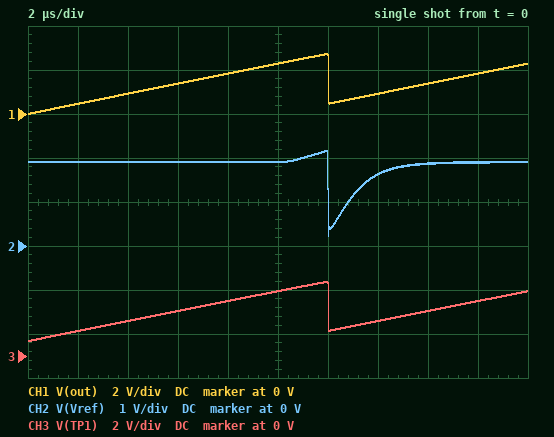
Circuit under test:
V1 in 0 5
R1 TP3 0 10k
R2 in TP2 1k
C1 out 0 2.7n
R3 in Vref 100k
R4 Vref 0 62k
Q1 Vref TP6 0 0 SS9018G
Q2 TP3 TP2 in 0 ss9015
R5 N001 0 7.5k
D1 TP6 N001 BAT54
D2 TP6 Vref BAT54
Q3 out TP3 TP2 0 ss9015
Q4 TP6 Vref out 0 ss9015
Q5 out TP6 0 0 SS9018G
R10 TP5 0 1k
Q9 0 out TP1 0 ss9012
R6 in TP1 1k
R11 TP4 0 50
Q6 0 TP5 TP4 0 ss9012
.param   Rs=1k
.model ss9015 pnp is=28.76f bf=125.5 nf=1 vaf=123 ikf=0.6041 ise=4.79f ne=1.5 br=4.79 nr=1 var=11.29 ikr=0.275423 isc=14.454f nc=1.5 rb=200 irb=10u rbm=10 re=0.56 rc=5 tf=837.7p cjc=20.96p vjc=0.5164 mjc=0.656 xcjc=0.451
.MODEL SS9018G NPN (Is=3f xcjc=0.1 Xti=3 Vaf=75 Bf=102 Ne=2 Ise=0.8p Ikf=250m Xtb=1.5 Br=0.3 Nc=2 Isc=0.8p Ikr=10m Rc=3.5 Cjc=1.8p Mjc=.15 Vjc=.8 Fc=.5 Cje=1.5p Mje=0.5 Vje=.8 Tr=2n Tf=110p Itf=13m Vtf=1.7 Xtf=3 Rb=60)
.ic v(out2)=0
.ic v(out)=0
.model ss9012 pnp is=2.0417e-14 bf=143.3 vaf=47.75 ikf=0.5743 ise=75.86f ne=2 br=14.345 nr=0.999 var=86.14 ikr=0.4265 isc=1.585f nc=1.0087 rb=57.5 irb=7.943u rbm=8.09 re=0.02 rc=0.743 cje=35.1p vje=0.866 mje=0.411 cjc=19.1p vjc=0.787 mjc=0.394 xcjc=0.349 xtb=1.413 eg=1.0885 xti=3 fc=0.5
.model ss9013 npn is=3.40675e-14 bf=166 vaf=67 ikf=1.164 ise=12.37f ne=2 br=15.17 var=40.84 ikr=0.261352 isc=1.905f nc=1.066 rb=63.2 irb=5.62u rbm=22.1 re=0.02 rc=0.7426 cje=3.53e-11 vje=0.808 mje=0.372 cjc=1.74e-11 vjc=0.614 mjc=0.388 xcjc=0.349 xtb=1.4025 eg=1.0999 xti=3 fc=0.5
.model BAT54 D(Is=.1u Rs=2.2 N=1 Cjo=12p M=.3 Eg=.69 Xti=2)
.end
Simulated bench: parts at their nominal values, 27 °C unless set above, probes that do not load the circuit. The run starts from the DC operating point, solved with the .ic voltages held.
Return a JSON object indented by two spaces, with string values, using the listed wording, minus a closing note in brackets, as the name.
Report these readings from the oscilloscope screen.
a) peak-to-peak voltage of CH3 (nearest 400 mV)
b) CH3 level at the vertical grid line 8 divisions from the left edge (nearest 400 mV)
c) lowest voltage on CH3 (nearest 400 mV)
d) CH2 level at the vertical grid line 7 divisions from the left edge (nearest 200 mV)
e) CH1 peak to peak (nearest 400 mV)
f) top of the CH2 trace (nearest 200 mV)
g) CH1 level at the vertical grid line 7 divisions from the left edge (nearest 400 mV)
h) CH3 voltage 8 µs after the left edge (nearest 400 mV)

{
  "peak-to-peak voltage of CH3": "2.8 V",
  "CH3 level at the vertical grid line 8 divisions from the left edge": "2.0 V",
  "lowest voltage on CH3": "800 mV",
  "CH2 level at the vertical grid line 7 divisions from the left edge": "1.6 V",
  "CH1 peak to peak": "2.8 V",
  "top of the CH2 trace": "2.2 V",
  "CH1 level at the vertical grid line 7 divisions from the left edge": "800 mV",
  "CH3 voltage 8 µs after the left edge": "2.4 V"
}
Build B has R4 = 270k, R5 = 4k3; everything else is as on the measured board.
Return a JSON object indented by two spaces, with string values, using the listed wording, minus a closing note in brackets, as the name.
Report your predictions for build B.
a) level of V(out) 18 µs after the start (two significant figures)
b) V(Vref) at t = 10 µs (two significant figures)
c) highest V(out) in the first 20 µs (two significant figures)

{
  "level of V(out) 18 µs after the start": "4.1 V",
  "V(Vref) at t = 10 µs": "3.6 V",
  "highest V(out) in the first 20 µs": "4.4 V"
}
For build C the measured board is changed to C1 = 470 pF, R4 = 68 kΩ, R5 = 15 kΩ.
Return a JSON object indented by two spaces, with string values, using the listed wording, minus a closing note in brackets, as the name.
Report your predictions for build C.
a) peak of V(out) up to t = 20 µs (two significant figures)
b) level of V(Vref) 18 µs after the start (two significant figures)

{
  "peak of V(out) up to t = 20 µs": "3.0 V",
  "level of V(Vref) 18 µs after the start": "450 mV"
}
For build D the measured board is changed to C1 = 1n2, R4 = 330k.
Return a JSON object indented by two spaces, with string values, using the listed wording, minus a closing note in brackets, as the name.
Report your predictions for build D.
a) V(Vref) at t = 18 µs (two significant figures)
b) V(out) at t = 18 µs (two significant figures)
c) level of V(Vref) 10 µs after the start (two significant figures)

{
  "V(Vref) at t = 18 µs": "3.8 V",
  "V(out) at t = 18 µs": "3.5 V",
  "level of V(Vref) 10 µs after the start": "4.0 V"
}
